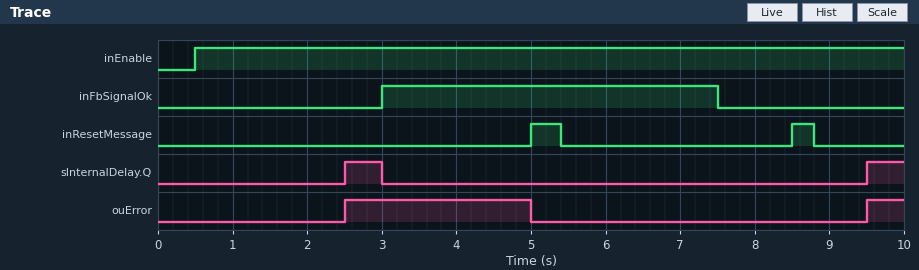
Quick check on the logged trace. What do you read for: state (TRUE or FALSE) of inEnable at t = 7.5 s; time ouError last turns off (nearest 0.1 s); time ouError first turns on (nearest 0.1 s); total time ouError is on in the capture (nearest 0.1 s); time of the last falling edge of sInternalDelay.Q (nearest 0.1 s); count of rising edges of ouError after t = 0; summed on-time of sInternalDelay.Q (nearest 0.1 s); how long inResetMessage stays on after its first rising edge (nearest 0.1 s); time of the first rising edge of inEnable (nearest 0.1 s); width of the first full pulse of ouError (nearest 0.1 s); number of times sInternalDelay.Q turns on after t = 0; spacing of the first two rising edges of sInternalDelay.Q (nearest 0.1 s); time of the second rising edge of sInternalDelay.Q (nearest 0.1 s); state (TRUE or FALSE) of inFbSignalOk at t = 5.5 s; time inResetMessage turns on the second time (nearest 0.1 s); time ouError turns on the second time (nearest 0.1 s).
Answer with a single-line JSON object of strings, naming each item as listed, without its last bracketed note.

{"state (TRUE or FALSE) of inEnable at t = 7.5 s": "TRUE", "time ouError last turns off": "5.0 s", "time ouError first turns on": "2.5 s", "total time ouError is on in the capture": "3.0 s", "time of the last falling edge of sInternalDelay.Q": "3.0 s", "count of rising edges of ouError after t = 0": "2", "summed on-time of sInternalDelay.Q": "1.0 s", "how long inResetMessage stays on after its first rising edge": "0.4 s", "time of the first rising edge of inEnable": "0.5 s", "width of the first full pulse of ouError": "2.5 s", "number of times sInternalDelay.Q turns on after t = 0": "2", "spacing of the first two rising edges of sInternalDelay.Q": "7.0 s", "time of the second rising edge of sInternalDelay.Q": "9.5 s", "state (TRUE or FALSE) of inFbSignalOk at t = 5.5 s": "TRUE", "time inResetMessage turns on the second time": "8.5 s", "time ouError turns on the second time": "9.5 s"}
